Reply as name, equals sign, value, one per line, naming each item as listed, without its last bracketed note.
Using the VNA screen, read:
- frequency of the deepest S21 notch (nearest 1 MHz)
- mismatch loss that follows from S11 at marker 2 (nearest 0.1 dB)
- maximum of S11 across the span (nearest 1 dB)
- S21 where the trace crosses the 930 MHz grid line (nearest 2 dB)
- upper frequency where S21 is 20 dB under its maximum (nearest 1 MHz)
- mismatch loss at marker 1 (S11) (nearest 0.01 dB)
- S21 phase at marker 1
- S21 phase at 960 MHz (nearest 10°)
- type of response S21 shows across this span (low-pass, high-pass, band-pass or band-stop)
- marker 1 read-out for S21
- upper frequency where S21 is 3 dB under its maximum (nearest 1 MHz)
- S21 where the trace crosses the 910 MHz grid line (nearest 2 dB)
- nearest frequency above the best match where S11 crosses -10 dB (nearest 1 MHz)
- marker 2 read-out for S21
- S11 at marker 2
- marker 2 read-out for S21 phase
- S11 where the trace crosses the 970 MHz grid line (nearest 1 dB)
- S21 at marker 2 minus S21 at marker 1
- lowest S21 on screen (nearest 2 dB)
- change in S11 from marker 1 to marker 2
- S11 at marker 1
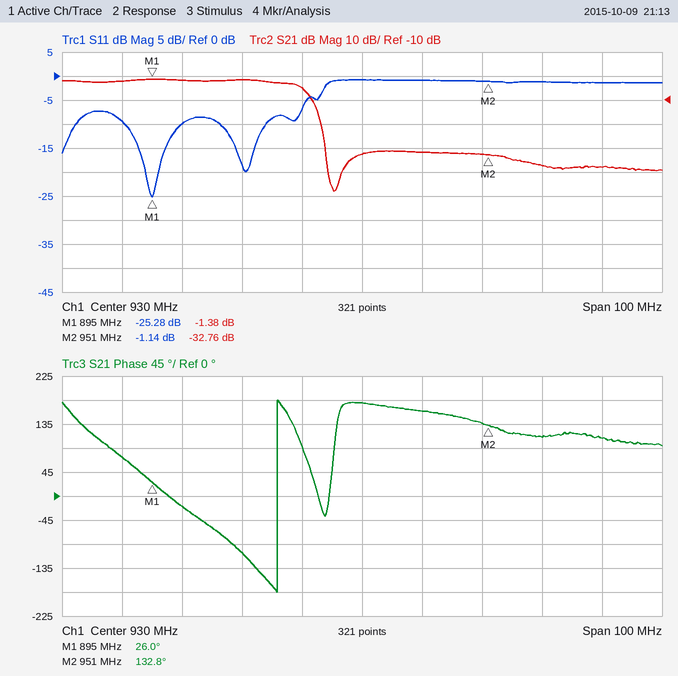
frequency of the deepest S21 notch = 925 MHz
mismatch loss that follows from S11 at marker 2 = 6.4 dB
maximum of S11 across the span = -1 dB
S21 where the trace crosses the 930 MHz grid line = -32 dB
upper frequency where S21 is 20 dB under its maximum = 923 MHz
mismatch loss at marker 1 (S11) = 0.01 dB
S21 phase at marker 1 = 26.0°
S21 phase at 960 MHz = 110°
type of response S21 shows across this span = low-pass
marker 1 read-out for S21 = -1.38 dB
upper frequency where S21 is 3 dB under its maximum = 920 MHz
S21 where the trace crosses the 910 MHz grid line = -2 dB
nearest frequency above the best match where S11 crosses -10 dB = 900 MHz
marker 2 read-out for S21 = -32.76 dB
S11 at marker 2 = -1.14 dB
marker 2 read-out for S21 phase = 132.8°
S11 where the trace crosses the 970 MHz grid line = -1 dB
S21 at marker 2 minus S21 at marker 1 = -31.38 dB
lowest S21 on screen = -48 dB
change in S11 from marker 1 to marker 2 = 24.14 dB
S11 at marker 1 = -25.28 dB
